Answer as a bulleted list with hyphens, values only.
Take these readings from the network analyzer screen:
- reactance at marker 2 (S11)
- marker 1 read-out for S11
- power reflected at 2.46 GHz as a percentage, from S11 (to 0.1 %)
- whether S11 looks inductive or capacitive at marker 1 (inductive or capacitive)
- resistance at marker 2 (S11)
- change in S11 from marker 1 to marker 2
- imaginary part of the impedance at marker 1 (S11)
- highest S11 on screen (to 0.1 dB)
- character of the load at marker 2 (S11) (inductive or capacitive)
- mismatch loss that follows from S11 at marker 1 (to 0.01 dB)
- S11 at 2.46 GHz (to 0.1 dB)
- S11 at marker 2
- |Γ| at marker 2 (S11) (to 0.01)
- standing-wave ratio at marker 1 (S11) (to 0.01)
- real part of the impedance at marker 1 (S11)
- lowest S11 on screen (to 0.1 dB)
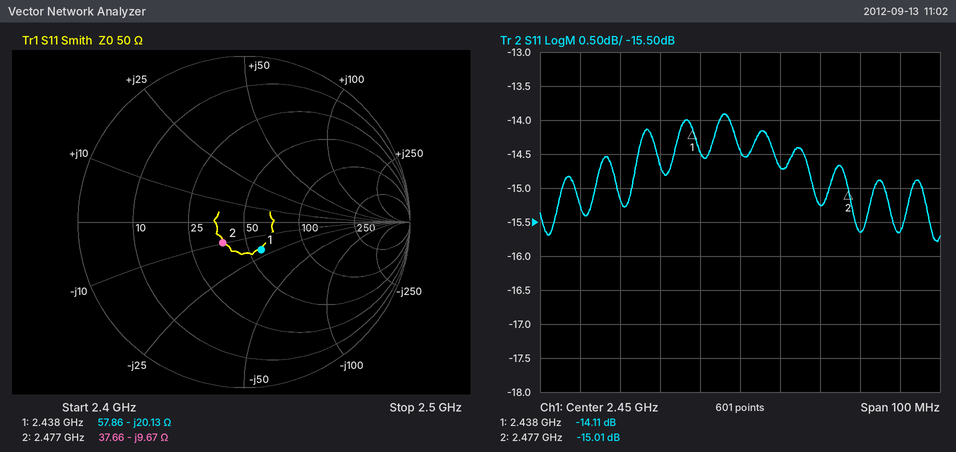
- -9.67 Ω
- -14.11 dB
- 3.4 %
- capacitive
- 37.66 Ω
- -0.90 dB
- -20.13 Ω
- -13.9 dB
- capacitive
- 0.17 dB
- -14.7 dB
- -15.01 dB
- 0.18
- 1.49
- 57.86 Ω
- -15.8 dB
